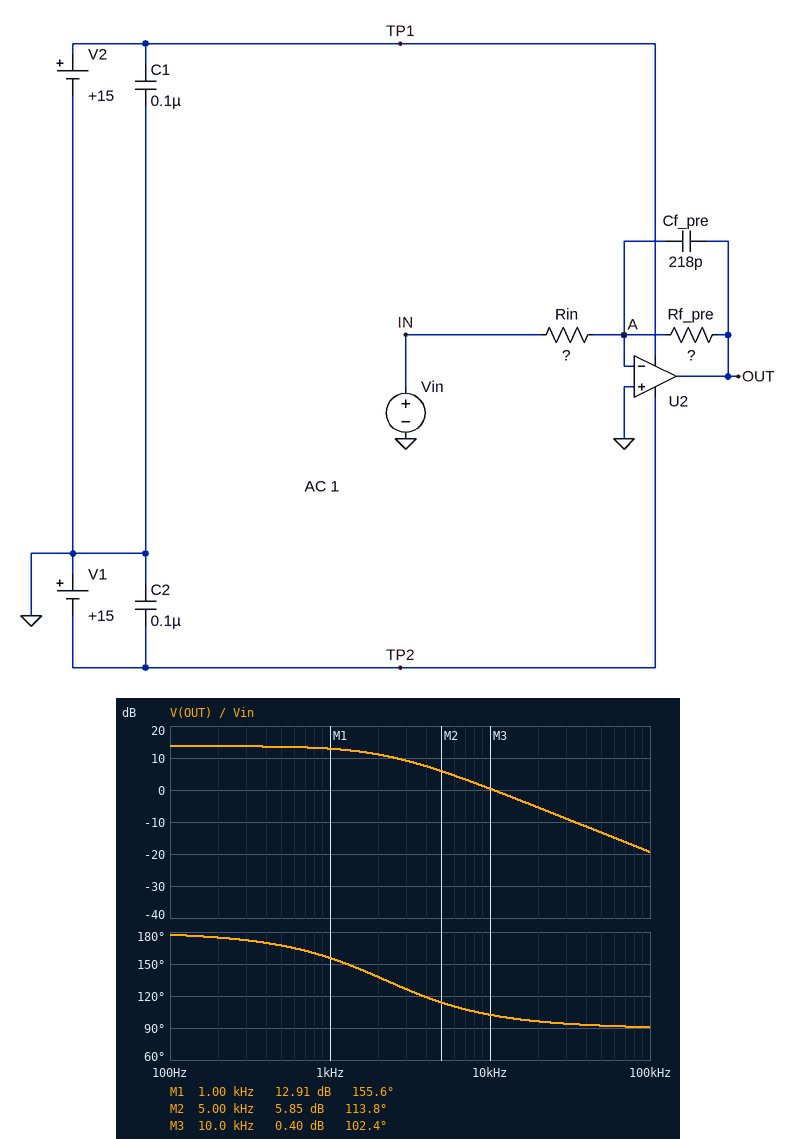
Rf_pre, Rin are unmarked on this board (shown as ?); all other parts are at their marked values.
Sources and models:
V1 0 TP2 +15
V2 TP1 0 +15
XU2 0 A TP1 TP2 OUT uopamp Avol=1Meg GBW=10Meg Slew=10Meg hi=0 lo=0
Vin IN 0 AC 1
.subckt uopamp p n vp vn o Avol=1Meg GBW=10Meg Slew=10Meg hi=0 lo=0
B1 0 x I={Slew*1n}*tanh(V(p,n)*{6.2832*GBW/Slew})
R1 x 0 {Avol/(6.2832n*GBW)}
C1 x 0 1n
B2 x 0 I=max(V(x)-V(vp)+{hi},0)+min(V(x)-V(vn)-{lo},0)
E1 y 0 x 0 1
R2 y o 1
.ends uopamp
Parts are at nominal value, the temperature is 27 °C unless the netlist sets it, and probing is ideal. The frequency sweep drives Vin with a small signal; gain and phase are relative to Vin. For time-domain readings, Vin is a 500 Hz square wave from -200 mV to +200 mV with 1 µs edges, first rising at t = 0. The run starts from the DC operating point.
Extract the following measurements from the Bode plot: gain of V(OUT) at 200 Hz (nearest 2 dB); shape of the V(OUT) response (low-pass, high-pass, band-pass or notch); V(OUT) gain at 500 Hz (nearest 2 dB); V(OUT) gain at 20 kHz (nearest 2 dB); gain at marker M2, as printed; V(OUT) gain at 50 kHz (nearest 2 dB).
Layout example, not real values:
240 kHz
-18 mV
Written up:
14 dB
low-pass
14 dB
-6 dB
5.85 dB
-14 dB
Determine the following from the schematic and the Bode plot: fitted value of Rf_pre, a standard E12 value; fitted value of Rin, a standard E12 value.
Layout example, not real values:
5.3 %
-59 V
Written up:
330 kΩ
68 kΩ
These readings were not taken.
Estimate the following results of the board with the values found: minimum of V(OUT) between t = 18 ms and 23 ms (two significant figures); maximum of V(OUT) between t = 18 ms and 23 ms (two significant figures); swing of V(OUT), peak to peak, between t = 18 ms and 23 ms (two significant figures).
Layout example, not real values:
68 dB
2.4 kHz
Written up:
-970 mV
970 mV
1.9 V
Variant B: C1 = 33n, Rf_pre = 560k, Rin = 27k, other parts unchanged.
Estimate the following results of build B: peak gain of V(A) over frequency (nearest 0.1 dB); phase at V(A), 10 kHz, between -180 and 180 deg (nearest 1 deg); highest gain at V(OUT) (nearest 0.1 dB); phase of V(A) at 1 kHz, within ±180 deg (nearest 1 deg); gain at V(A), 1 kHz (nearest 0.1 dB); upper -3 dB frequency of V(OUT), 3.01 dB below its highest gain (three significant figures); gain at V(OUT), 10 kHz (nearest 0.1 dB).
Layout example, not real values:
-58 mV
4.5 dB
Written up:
-51.4 dB
7 deg
26.3 dB
52 deg
-55.7 dB
1.30 kHz
8.5 dB
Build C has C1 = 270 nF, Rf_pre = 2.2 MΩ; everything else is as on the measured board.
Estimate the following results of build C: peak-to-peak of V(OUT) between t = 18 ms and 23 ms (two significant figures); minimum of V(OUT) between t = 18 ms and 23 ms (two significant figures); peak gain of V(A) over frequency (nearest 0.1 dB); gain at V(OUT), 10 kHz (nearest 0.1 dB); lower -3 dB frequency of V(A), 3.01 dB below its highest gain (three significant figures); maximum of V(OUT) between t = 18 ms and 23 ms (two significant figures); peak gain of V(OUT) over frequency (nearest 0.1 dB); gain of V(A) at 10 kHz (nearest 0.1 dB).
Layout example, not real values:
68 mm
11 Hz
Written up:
10 V
-5.0 V
-59.4 dB
0.6 dB
331 Hz
5.0 V
30.2 dB
-59.4 dB
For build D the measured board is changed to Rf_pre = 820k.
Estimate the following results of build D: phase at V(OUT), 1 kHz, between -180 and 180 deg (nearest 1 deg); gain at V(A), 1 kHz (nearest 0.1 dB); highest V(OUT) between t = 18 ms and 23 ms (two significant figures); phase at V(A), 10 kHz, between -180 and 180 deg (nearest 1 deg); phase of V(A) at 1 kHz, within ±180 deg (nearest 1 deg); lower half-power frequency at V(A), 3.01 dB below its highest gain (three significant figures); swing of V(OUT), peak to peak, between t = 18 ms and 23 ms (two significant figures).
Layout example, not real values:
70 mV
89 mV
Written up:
132 deg
-61.9 dB
2.4 V
5 deg
41 deg
889 Hz
4.8 V
